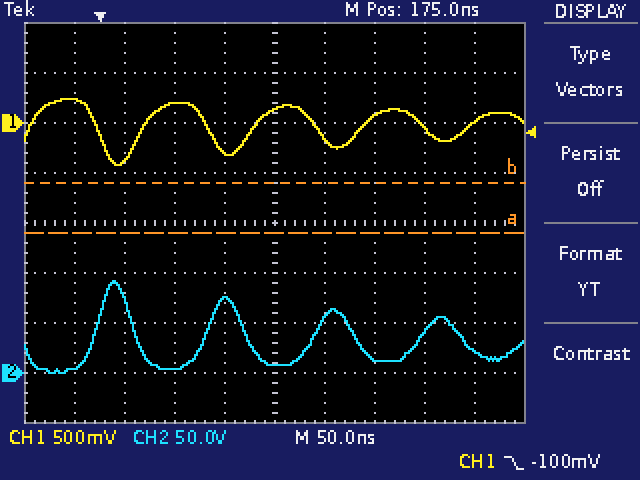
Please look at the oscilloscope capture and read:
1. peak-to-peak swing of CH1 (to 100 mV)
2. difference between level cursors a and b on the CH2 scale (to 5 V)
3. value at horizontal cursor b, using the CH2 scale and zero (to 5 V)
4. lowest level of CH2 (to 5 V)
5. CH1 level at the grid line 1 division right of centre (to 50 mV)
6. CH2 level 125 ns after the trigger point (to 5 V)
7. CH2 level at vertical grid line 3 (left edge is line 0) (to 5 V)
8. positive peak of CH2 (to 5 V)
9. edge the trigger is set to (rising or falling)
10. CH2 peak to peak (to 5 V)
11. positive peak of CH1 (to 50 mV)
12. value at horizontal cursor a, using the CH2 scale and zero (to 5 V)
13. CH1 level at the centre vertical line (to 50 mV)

700 mV
50 V
190 V
0 V
-150 mV
75 V
5 V
90 V
falling
90 V
250 mV
140 V
150 mV
